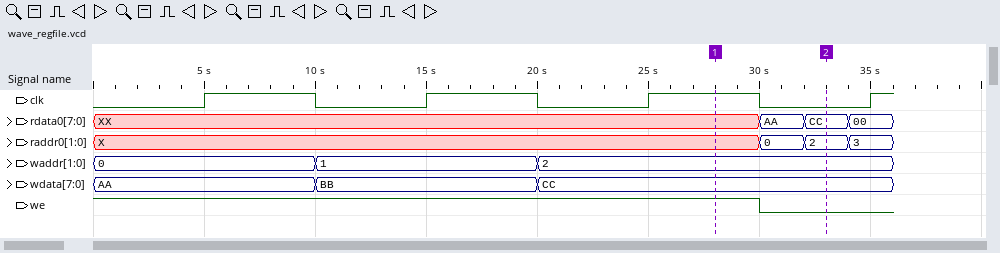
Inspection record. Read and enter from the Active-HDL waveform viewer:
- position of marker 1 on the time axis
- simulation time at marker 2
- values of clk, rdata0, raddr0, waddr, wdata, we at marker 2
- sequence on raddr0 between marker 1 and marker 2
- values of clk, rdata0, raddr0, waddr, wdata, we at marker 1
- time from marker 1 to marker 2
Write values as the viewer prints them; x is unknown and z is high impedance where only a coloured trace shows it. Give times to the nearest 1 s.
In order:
28 s
33 s
clk=0, rdata0=CC, raddr0=2, waddr=2, wdata=CC, we=0
X, 0, 2
clk=1, rdata0=XX, raddr0=X, waddr=2, wdata=CC, we=1
5 s
